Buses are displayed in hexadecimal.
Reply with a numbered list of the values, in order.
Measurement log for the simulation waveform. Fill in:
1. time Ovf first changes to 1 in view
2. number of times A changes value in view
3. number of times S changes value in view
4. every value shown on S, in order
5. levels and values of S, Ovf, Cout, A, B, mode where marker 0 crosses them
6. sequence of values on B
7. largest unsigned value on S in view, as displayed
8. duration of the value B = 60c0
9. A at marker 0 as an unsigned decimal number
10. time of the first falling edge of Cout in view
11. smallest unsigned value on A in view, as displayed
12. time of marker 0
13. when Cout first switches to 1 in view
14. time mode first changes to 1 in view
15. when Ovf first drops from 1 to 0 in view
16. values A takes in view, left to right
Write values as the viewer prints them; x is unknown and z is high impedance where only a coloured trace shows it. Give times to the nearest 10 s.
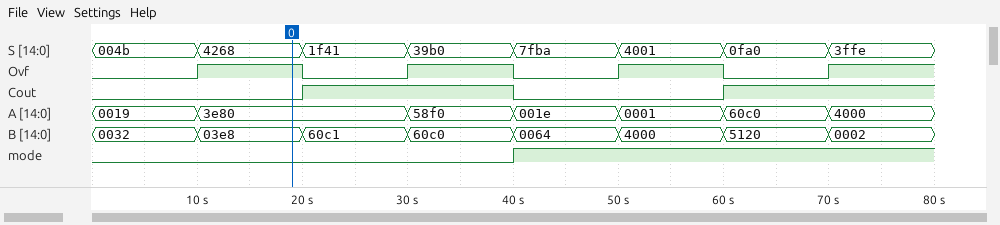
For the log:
1. 10 s
2. 6
3. 7
4. 004b, 4268, 1f41, 39b0, 7fba, 4001, 0fa0, 3ffe
5. S=4268, Ovf=1, Cout=0, A=3e80, B=03e8, mode=0
6. 0032, 03e8, 60c1, 60c0, 0064, 4000, 5120, 0002
7. 7fba
8. 10 s
9. 16000
10. 40 s
11. 0001
12. 20 s
13. 20 s
14. 40 s
15. 20 s
16. 0019, 3e80, 58f0, 001e, 0001, 60c0, 4000
